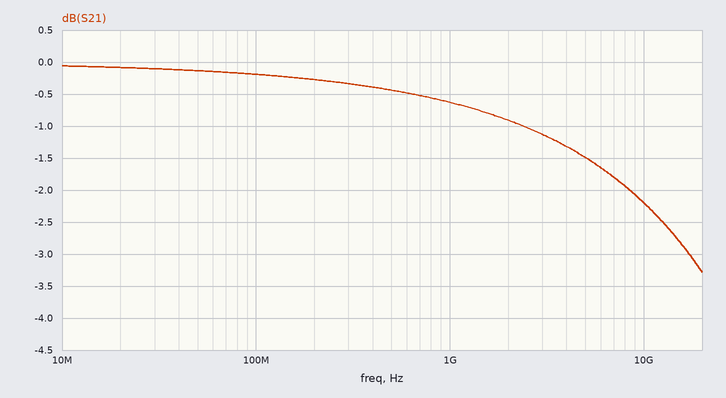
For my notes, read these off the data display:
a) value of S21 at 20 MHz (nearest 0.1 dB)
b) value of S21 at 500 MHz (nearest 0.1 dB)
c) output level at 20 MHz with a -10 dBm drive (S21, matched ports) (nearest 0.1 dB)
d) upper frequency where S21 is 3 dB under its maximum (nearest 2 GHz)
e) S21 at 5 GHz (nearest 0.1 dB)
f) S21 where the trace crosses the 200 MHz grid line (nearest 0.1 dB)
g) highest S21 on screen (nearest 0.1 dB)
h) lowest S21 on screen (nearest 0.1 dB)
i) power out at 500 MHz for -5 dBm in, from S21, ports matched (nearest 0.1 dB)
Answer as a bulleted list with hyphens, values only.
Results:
- -0.1 dB
- -0.4 dB
- -10.1 dBm
- 18 GHz
- -1.5 dB
- -0.3 dB
- -0.1 dB
- -3.3 dB
- -5.4 dBm
